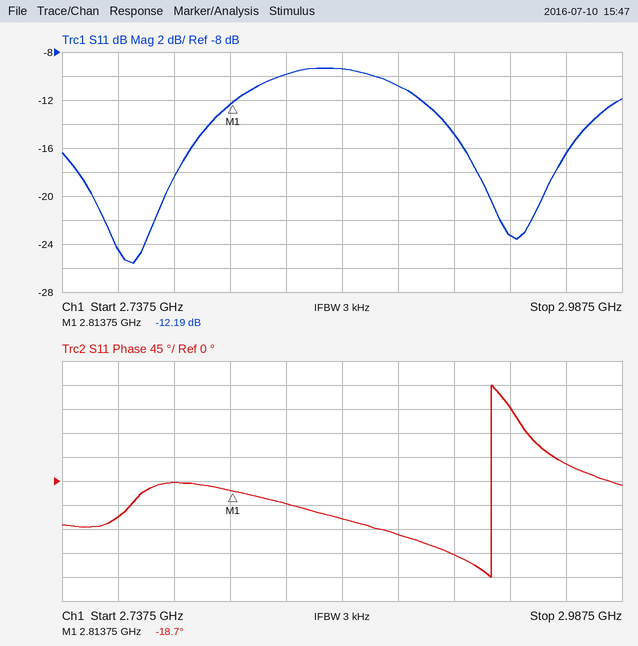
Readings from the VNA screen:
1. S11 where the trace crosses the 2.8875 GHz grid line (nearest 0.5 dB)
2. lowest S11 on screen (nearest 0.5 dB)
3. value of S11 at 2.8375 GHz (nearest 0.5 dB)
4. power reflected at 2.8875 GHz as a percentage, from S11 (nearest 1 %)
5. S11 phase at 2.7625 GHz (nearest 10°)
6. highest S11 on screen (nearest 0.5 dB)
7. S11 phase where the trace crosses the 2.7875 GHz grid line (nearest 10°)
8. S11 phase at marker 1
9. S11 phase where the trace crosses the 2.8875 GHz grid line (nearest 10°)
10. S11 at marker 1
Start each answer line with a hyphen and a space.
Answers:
- -11.0 dB
- -25.5 dB
- -10.0 dB
- 8 %
- -70°
- -9.5 dB
- 0°
- -18.7°
- -100°
- -12.19 dB
